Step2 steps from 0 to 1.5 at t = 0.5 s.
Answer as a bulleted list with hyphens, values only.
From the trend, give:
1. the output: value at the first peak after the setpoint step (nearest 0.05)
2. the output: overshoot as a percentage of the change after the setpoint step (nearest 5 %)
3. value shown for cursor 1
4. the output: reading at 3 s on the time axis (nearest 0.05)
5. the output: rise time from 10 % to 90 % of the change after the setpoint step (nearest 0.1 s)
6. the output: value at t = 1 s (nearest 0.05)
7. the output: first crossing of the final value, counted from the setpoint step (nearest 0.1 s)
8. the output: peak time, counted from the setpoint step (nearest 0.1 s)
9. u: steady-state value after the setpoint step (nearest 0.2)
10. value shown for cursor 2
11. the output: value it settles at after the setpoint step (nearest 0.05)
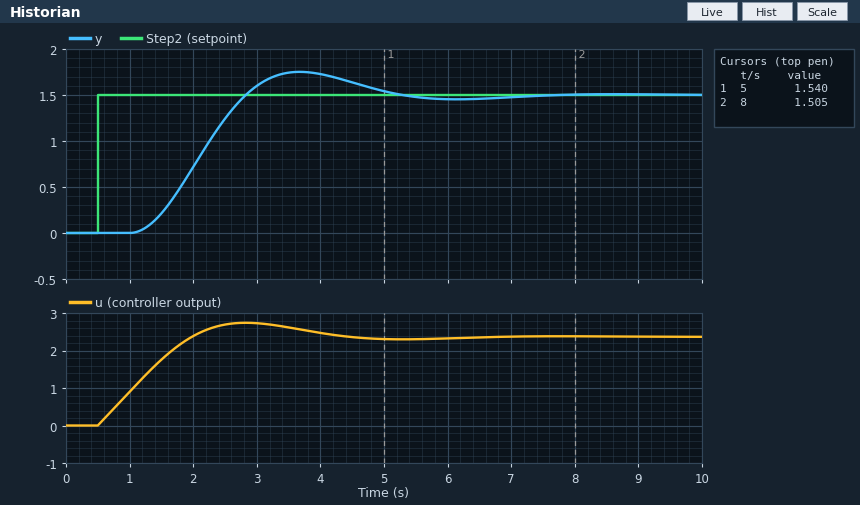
- 1.75
- 15 %
- 1.540
- 1.60
- 1.2 s
- 0.00
- 2.3 s
- 3.2 s
- 2.4
- 1.505
- 1.50
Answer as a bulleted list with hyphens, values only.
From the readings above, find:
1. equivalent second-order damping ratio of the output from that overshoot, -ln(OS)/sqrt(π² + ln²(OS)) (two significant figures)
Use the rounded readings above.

- 0.52
